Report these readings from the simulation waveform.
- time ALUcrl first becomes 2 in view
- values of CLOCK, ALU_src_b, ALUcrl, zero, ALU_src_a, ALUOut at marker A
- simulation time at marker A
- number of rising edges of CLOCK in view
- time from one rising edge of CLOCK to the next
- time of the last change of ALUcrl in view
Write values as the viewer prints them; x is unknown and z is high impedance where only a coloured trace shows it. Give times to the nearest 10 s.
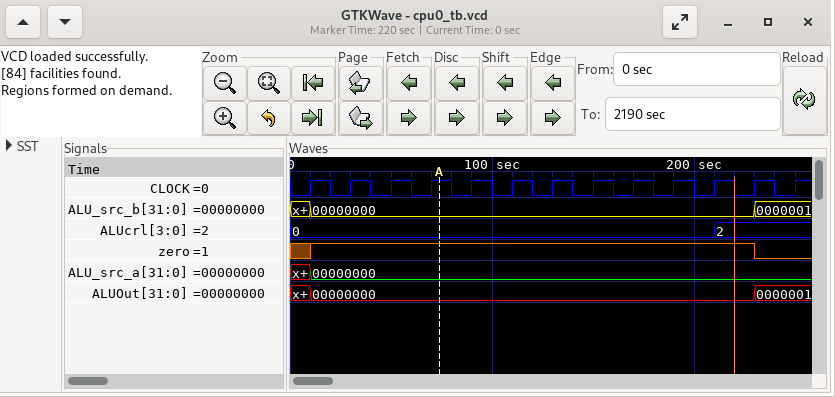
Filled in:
210 s
CLOCK=1, ALU_src_b=00000000, ALUcrl=0, zero=1, ALU_src_a=00000000, ALUOut=00000000
70 s
13
20 s
210 s
